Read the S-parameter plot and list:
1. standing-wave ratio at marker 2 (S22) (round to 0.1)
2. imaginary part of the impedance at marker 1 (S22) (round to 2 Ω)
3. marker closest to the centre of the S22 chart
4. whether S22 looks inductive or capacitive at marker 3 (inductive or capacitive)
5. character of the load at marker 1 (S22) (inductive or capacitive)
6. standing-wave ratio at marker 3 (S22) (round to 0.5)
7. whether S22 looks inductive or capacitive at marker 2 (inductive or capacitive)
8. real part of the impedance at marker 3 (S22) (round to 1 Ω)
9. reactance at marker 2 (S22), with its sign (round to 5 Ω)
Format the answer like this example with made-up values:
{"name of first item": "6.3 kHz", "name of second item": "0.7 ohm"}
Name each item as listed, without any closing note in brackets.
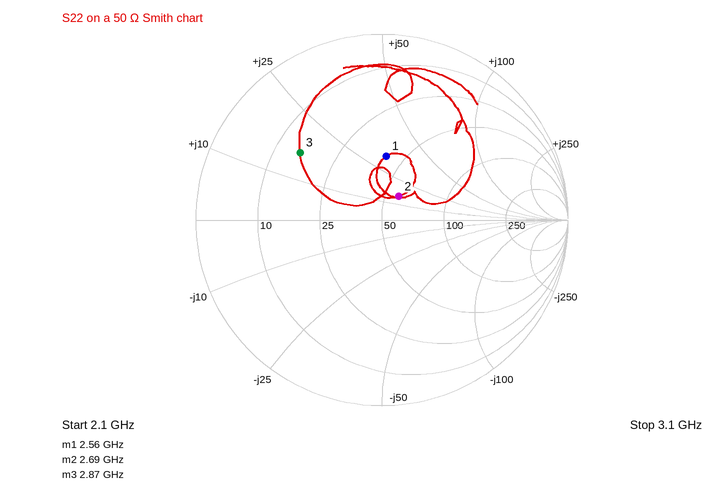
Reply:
{"standing-wave ratio at marker 2 (S22)": "1.4", "imaginary part of the impedance at marker 1 (S22)": "+32 Ω", "marker closest to the centre of the S22 chart": "marker 2", "whether S22 looks inductive or capacitive at marker 3": "inductive", "character of the load at marker 1 (S22)": "inductive", "standing-wave ratio at marker 3 (S22)": "3.5", "whether S22 looks inductive or capacitive at marker 2": "inductive", "real part of the impedance at marker 3 (S22)": "15 Ω", "reactance at marker 2 (S22), with its sign": "+15 Ω"}
